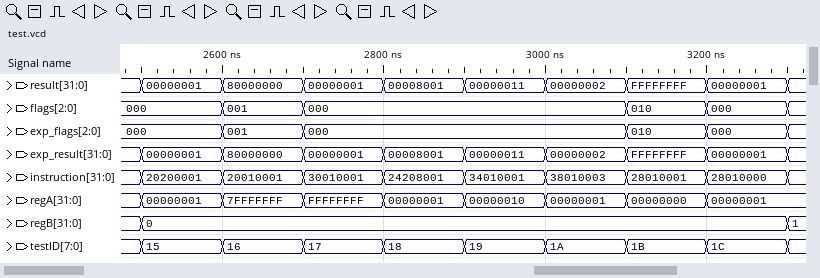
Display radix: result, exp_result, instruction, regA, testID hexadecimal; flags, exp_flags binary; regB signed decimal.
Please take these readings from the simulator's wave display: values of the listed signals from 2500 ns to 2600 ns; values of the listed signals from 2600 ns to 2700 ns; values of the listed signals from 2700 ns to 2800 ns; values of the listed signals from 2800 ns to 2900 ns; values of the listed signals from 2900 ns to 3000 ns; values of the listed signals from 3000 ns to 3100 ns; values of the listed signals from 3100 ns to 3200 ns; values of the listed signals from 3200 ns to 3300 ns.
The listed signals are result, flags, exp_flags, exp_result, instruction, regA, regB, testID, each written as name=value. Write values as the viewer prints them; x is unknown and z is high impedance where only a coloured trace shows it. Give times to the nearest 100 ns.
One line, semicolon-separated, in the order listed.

result=00000001, flags=000, exp_flags=000, exp_result=00000001, instruction=20200001, regA=00000001, regB=0, testID=15; result=80000000, flags=001, exp_flags=001, exp_result=80000000, instruction=20010001, regA=7FFFFFFF, regB=0, testID=16; result=00000001, flags=000, exp_flags=000, exp_result=00000001, instruction=30010001, regA=FFFFFFFF, regB=0, testID=17; result=00008001, flags=000, exp_flags=000, exp_result=00008001, instruction=24208001, regA=00000001, regB=0, testID=18; result=00000011, flags=000, exp_flags=000, exp_result=00000011, instruction=34010001, regA=00000010, regB=0, testID=19; result=00000002, flags=000, exp_flags=000, exp_result=00000002, instruction=38010003, regA=00000001, regB=0, testID=1A; result=FFFFFFFF, flags=010, exp_flags=010, exp_result=FFFFFFFF, instruction=28010001, regA=00000000, regB=0, testID=1B; result=00000001, flags=000, exp_flags=000, exp_result=00000001, instruction=28010000, regA=00000001, regB=0, testID=1C
